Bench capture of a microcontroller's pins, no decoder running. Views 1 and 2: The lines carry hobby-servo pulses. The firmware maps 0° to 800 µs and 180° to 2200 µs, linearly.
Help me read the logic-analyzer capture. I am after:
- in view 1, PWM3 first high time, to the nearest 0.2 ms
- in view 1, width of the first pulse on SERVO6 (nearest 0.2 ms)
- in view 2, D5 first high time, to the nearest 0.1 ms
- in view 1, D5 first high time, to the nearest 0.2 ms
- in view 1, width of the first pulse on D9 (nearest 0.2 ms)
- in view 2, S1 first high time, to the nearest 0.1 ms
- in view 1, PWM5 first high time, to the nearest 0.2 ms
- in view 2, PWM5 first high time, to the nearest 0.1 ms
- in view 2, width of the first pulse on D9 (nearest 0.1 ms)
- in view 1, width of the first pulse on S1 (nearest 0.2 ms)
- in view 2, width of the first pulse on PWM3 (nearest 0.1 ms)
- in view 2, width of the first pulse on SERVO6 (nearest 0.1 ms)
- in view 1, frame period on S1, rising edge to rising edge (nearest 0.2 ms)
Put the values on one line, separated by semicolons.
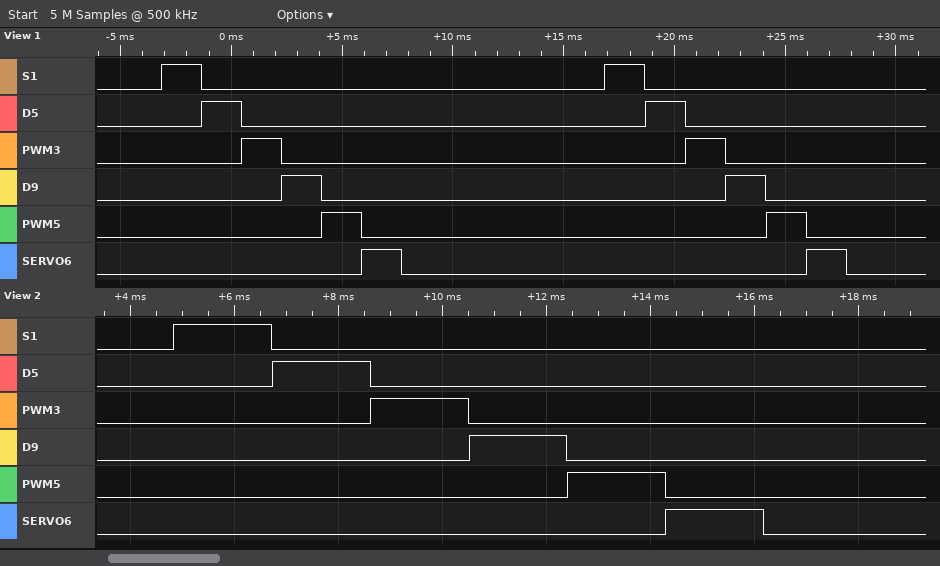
1.8 ms; 1.8 ms; 1.9 ms; 1.8 ms; 1.8 ms; 1.9 ms; 1.8 ms; 1.9 ms; 1.9 ms; 1.8 ms; 1.9 ms; 1.9 ms; 20.0 ms
